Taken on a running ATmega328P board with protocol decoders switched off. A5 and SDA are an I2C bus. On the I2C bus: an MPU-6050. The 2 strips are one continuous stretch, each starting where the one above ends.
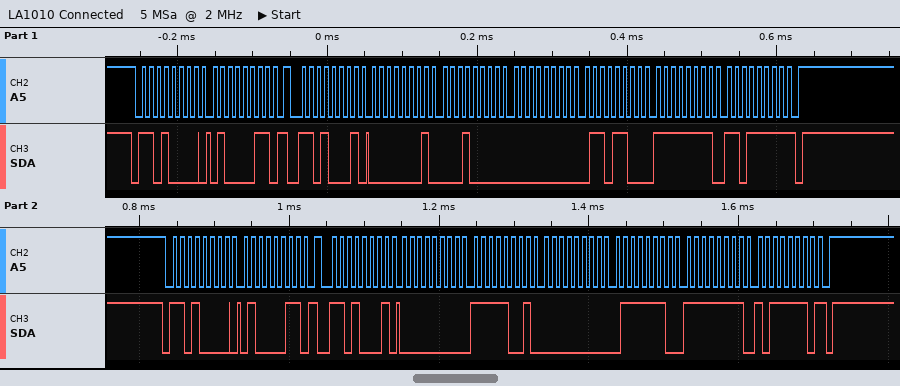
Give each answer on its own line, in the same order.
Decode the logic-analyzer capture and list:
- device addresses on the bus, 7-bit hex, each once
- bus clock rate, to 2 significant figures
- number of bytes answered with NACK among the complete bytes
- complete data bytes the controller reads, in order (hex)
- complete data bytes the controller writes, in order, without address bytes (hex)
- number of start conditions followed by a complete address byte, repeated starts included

0x68
100 kHz
2
01 10 00 6C FF DF 00 F9 00 7E FF BE
43 43
4
